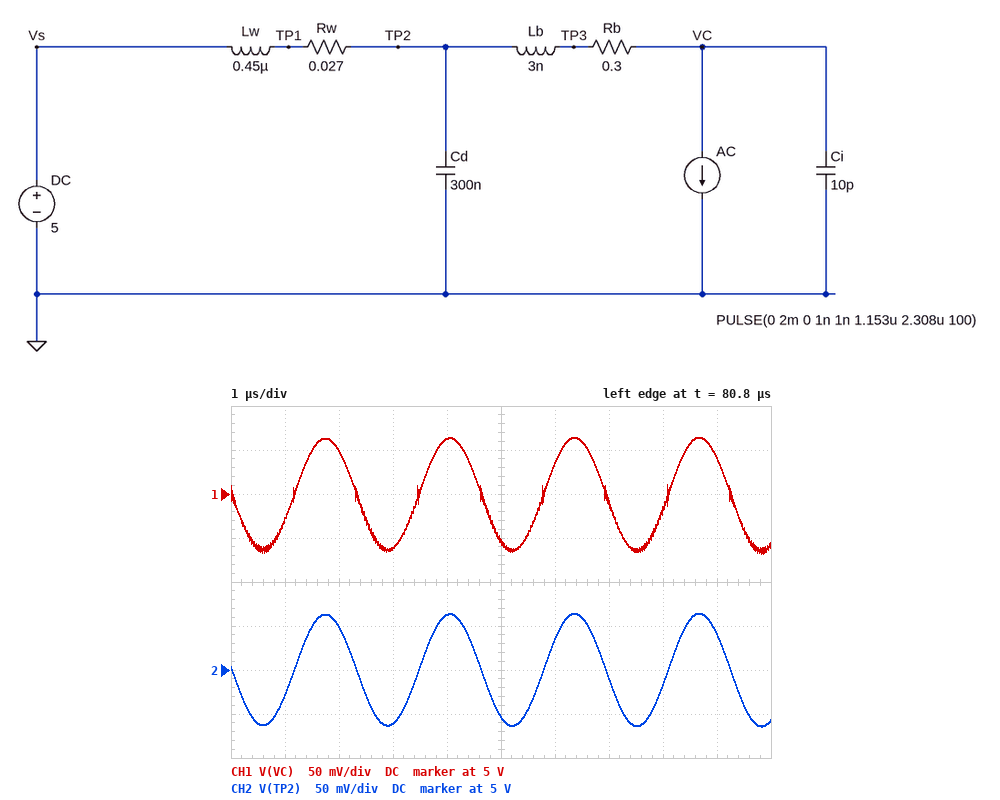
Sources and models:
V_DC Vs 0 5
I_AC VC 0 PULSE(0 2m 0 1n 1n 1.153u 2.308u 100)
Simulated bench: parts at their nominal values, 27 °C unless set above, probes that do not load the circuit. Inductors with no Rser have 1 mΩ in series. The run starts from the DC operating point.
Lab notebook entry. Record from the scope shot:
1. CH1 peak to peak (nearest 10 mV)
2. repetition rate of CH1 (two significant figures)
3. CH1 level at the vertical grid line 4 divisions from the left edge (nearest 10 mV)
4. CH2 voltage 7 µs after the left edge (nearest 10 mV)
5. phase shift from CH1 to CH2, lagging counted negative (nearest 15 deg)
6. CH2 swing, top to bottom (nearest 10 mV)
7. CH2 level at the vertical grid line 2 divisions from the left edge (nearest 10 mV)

130 mV
430 kHz
5.06 V
4.99 V
0 deg
130 mV
5.05 V
